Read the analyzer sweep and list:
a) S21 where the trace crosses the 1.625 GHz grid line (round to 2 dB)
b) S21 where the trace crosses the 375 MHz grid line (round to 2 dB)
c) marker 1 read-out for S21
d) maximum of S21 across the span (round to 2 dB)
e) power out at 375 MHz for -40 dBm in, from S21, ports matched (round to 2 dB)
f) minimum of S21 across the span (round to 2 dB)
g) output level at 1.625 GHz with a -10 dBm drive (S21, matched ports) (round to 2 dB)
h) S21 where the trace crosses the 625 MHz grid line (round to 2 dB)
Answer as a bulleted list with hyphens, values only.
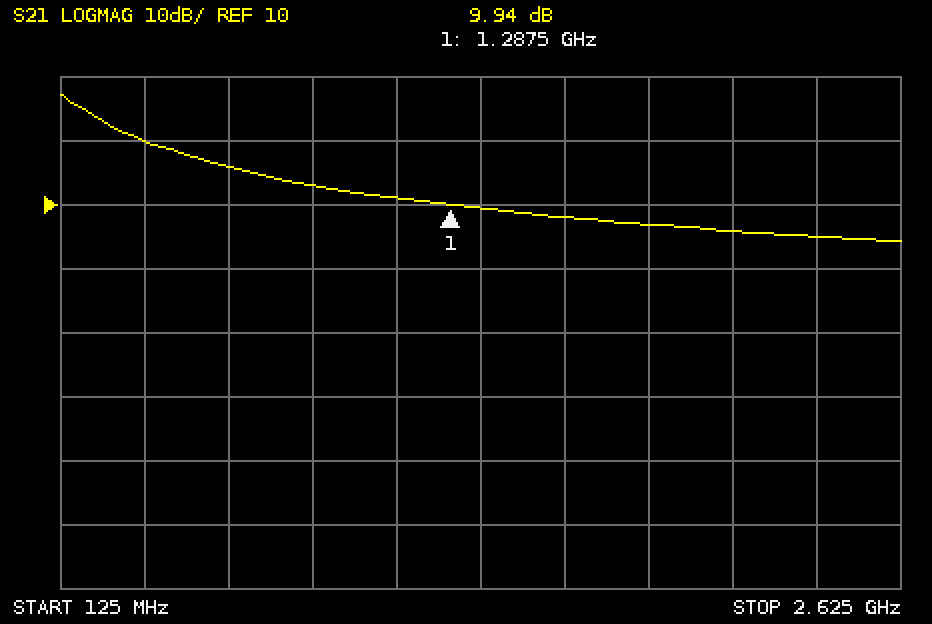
- 8 dB
- 20 dB
- 9.94 dB
- 28 dB
- -20 dBm
- 4 dB
- -2 dBm
- 16 dB
